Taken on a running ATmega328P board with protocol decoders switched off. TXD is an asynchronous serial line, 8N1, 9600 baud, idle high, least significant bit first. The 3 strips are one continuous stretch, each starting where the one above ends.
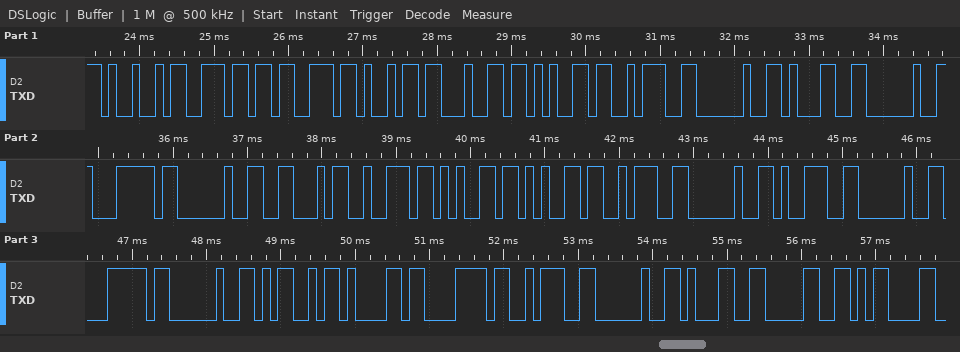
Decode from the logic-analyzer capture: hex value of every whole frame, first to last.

0x49 0x6E 0x73 0x69 0x64 0x65 0x3A 0x20 0x31 0x20 0x7C 0x20 0x46 0x72 0x65 0x65 0x3A 0x20 0x39 0x20 0x7C 0x20 0x4D 0x61 0x78 0x3A 0x20 0x31 0x30 0x0D
